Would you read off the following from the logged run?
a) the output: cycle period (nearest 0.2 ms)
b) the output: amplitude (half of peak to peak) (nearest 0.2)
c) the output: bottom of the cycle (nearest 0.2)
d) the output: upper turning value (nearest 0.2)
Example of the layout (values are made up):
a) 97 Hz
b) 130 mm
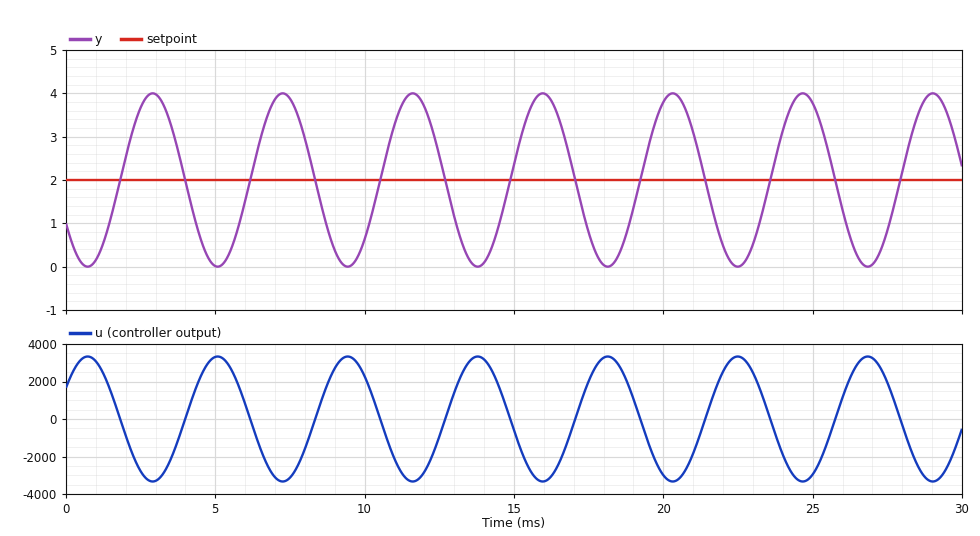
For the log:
a) 4.4 ms
b) 2.0
c) 0.0
d) 4.0
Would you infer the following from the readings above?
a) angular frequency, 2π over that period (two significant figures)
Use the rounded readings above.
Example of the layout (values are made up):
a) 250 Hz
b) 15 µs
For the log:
a) 1.4 rad/ms
